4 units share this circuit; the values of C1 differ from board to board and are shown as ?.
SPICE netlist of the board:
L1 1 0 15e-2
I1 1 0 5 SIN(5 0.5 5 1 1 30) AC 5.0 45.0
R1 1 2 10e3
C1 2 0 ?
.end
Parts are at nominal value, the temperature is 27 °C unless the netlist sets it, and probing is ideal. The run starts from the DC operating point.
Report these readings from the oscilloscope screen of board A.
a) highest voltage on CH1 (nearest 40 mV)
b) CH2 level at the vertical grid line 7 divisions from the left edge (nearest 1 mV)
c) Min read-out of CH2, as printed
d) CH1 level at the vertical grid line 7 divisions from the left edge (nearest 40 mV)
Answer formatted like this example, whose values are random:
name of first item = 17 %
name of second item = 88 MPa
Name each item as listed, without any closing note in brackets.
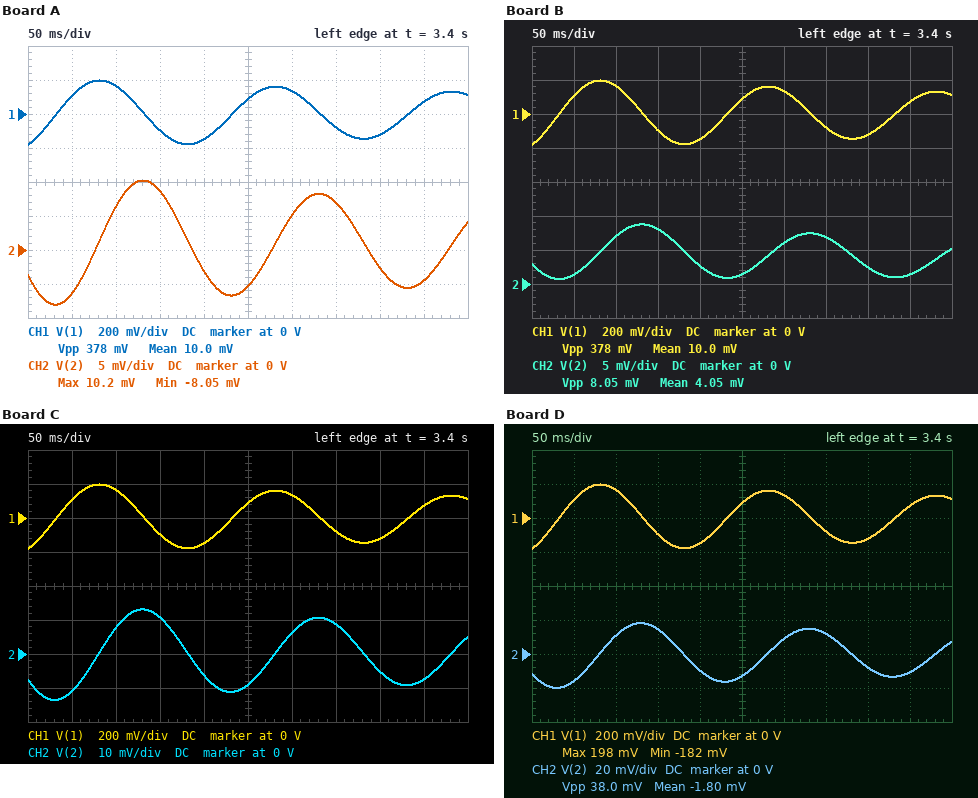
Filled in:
highest voltage on CH1 = 200 mV
CH2 level at the vertical grid line 7 divisions from the left edge = 7 mV
Min read-out of CH2, as printed = -8.05 mV
CH1 level at the vertical grid line 7 divisions from the left edge = -80 mV
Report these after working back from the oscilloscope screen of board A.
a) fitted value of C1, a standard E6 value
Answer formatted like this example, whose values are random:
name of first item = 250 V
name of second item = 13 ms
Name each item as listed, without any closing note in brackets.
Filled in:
fitted value of C1, a standard E6 value = 68 µF
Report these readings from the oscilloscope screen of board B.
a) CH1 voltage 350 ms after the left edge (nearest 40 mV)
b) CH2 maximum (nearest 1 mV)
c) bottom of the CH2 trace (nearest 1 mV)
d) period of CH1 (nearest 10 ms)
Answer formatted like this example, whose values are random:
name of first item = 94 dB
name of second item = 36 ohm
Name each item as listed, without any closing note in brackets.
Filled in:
CH1 voltage 350 ms after the left edge = -80 mV
CH2 maximum = 9 mV
bottom of the CH2 trace = 1 mV
period of CH1 = 200 ms
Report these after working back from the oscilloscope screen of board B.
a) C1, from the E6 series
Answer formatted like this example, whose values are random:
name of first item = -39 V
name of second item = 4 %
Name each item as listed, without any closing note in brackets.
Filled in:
C1, from the E6 series = 150 µF
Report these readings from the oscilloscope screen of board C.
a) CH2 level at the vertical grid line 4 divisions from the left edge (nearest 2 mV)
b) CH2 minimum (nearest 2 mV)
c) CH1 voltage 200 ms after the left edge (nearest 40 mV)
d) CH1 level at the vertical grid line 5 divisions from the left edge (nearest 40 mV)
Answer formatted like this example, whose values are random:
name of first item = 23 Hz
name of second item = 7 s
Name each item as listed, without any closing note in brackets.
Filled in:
CH2 level at the vertical grid line 4 divisions from the left edge = -6 mV
CH2 minimum = -14 mV
CH1 voltage 200 ms after the left edge = -160 mV
CH1 level at the vertical grid line 5 divisions from the left edge = 80 mV
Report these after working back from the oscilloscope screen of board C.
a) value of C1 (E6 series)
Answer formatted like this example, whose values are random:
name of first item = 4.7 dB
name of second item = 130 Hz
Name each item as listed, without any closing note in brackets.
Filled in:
value of C1 = 47 µF
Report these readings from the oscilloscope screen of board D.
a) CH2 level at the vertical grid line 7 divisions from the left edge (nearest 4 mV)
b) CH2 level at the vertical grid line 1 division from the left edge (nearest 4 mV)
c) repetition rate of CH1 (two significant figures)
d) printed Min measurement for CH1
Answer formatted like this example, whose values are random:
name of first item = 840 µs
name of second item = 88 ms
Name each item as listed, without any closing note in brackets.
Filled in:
CH2 level at the vertical grid line 7 divisions from the left edge = 12 mV
CH2 level at the vertical grid line 1 division from the left edge = -16 mV
repetition rate of CH1 = 5.0 Hz
printed Min measurement for CH1 = -182 mV
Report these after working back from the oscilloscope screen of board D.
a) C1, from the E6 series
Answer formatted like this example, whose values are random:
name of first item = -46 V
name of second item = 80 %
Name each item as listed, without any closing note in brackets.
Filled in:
C1, from the E6 series = 33 µF
